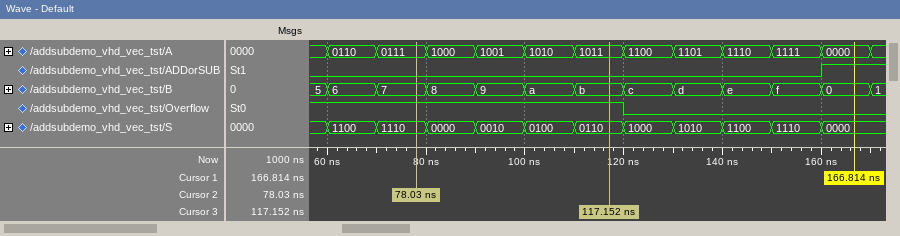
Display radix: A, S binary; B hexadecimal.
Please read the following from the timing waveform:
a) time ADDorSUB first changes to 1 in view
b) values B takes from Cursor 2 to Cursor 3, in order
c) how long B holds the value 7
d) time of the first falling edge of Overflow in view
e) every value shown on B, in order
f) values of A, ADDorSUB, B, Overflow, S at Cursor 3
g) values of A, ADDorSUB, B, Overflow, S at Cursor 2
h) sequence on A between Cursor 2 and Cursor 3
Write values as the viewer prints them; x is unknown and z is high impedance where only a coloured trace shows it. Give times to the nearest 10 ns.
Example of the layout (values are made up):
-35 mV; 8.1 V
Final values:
160 ns; 7, 8, 9, a, b; 10 ns; 120 ns; 5, 6, 7, 8, 9, a, b, c, d, e, f, 0, 1; A=1011, ADDorSUB=0, B=b, Overflow=1, S=0110; A=0111, ADDorSUB=0, B=7, Overflow=1, S=1110; 0111, 1000, 1001, 1010, 1011
